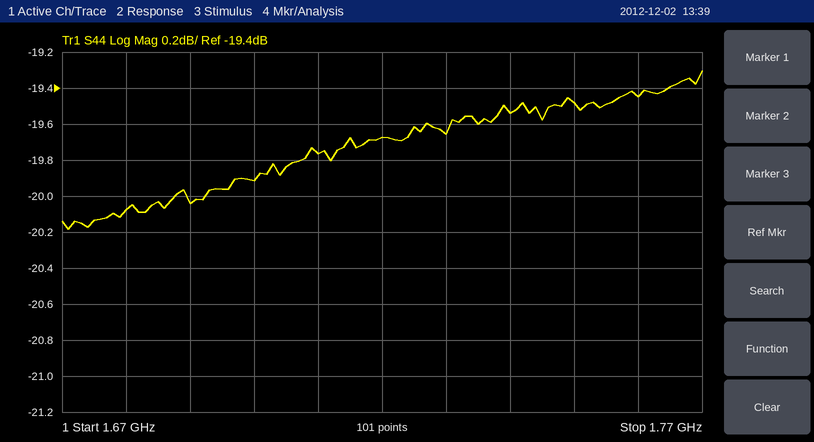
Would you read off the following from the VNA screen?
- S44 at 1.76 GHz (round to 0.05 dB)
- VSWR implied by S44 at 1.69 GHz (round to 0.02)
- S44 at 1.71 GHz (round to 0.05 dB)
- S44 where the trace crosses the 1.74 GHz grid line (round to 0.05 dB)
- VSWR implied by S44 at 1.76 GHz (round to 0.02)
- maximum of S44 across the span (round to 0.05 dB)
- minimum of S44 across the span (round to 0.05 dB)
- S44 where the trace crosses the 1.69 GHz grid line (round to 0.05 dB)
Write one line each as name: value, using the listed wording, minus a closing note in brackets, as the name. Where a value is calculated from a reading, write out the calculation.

S44 at 1.76 GHz: -19.45 dB
VSWR implied by S44 at 1.69 GHz: |Γ| = 10^(-20.05/20) = 0.0994; VSWR = (1 + 0.0994)/(1 − 0.0994) ≈ 1.22
S44 at 1.71 GHz: -19.75 dB
S44 where the trace crosses the 1.74 GHz grid line: -19.55 dB
VSWR implied by S44 at 1.76 GHz: |Γ| = 10^(-19.45/20) = 0.1065; VSWR = (1 + 0.1065)/(1 − 0.1065) ≈ 1.24
maximum of S44 across the span: -19.30 dB
minimum of S44 across the span: -20.20 dB
S44 where the trace crosses the 1.69 GHz grid line: -20.05 dB
